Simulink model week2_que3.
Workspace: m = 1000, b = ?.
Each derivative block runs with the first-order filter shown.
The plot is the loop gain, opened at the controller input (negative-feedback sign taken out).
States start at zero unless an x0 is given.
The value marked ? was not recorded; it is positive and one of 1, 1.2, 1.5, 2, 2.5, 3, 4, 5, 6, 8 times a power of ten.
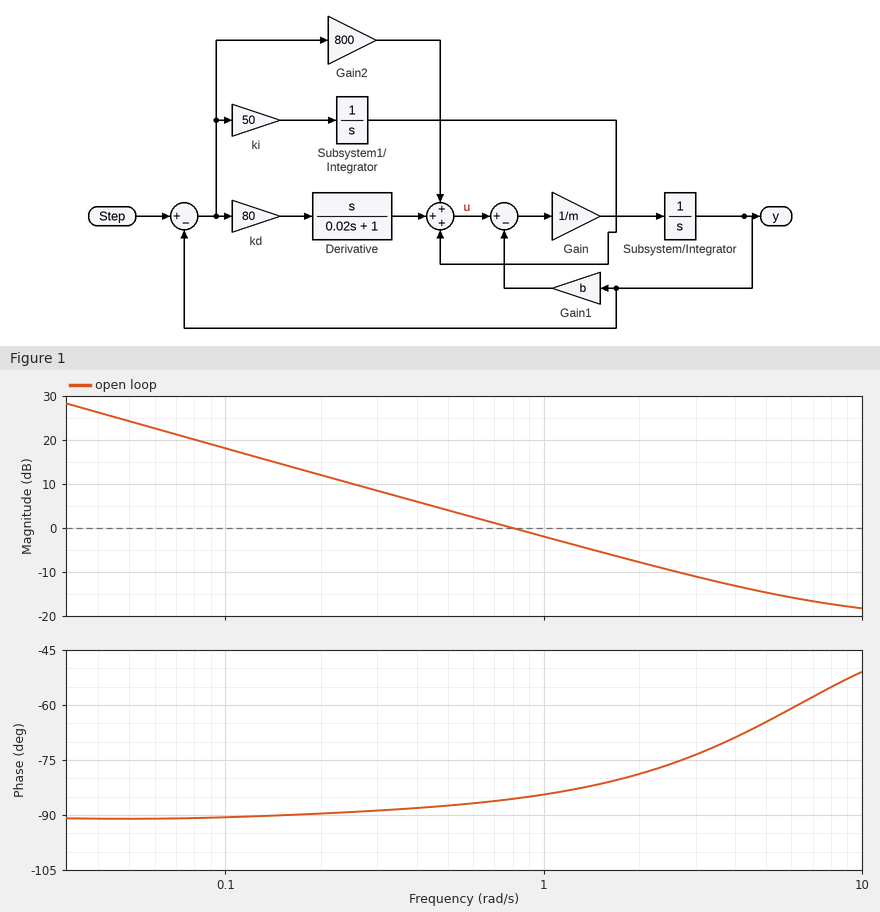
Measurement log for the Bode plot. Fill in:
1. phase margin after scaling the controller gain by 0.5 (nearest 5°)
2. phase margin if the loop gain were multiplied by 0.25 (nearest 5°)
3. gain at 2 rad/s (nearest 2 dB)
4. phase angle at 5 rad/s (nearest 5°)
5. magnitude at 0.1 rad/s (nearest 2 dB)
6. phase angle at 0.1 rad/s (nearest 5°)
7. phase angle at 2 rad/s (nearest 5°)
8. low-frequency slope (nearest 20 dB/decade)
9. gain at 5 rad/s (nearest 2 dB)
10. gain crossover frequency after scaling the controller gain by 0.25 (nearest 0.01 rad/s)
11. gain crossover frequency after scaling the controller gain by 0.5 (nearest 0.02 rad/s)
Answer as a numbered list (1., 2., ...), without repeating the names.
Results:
1. 90°
2. 90°
3. -8 dB
4. -65°
5. 18 dB
6. -90°
7. -80°
8. -20 dB/decade
9. -14 dB
10. 0.20 rad/s
11. 0.40 rad/s
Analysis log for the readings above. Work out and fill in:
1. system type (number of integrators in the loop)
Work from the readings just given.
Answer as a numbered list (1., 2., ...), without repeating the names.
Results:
1. 1
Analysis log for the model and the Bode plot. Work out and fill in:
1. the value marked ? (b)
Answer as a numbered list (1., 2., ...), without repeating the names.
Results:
1. 60
